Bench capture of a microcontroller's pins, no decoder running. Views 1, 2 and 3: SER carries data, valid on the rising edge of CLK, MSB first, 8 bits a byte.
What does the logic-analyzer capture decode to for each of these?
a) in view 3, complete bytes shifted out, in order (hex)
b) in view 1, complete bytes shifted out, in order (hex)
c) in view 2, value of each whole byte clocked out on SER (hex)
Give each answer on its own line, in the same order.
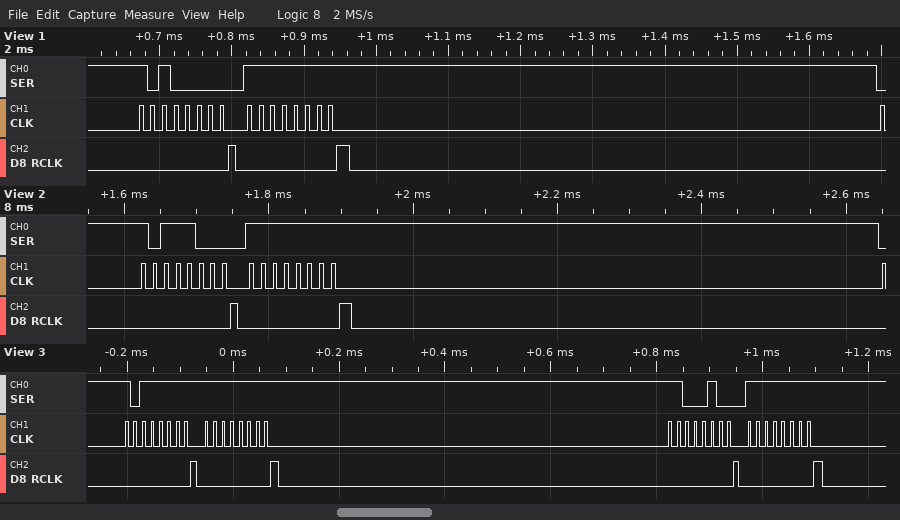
BF FF C4 FF
A0 FF
0xB8 0xFF
